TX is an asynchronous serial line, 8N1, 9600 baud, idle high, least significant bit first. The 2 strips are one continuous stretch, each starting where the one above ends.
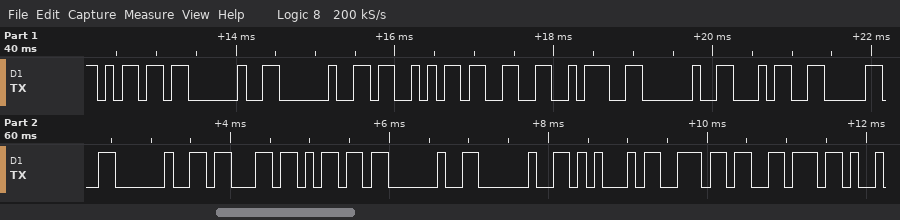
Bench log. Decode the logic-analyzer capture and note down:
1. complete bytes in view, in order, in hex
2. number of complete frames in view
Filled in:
6D 20 20 53 33 3A 20 34 30 20 63 6D 20 20 45 6E 76
17
